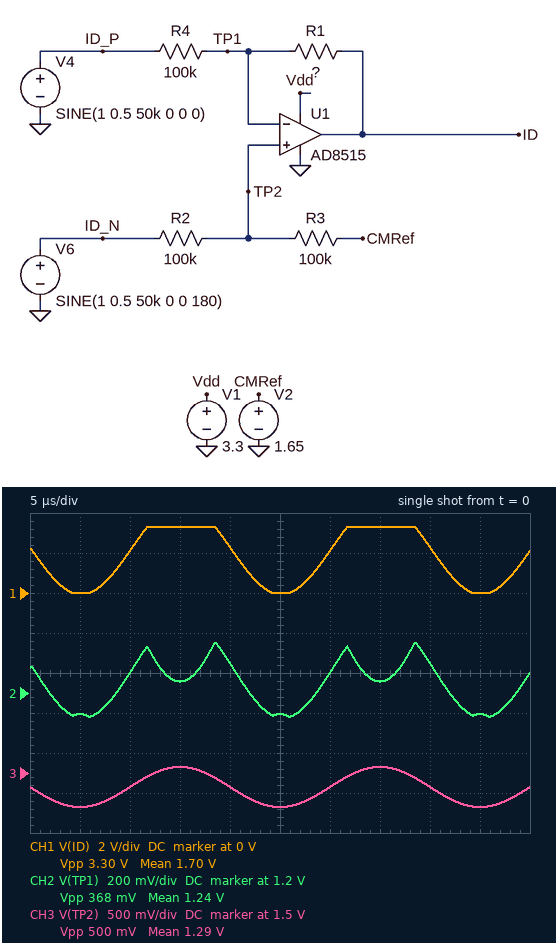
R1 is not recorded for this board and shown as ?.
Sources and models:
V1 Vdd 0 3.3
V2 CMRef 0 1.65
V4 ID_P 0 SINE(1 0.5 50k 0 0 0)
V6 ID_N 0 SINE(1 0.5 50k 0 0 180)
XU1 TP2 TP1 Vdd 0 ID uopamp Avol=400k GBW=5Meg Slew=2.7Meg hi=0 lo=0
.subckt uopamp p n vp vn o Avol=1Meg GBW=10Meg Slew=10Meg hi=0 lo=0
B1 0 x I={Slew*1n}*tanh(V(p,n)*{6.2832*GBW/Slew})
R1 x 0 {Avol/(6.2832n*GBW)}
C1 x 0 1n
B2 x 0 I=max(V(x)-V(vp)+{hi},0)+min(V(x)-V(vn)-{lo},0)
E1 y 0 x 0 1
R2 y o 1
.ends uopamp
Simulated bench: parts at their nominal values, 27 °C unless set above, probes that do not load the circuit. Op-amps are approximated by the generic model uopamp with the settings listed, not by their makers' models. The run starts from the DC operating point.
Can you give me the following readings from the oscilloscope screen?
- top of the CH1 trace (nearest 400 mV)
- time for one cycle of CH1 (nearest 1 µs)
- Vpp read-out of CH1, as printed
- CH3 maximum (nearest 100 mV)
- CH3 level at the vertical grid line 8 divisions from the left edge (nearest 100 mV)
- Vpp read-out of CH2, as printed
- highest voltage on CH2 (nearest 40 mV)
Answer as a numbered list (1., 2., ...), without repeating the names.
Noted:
1. 3.2 V
2. 20 µs
3. 3.30 V
4. 1.6 V
5. 1.3 V
6. 368 mV
7. 1.44 V
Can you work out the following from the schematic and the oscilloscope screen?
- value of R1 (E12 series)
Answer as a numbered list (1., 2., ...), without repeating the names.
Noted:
1. 270 kΩ
